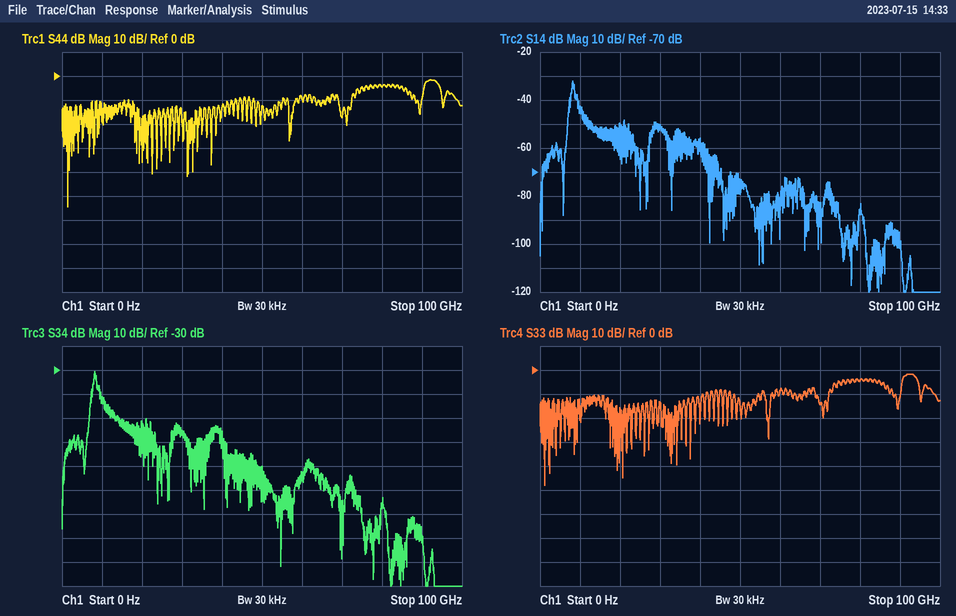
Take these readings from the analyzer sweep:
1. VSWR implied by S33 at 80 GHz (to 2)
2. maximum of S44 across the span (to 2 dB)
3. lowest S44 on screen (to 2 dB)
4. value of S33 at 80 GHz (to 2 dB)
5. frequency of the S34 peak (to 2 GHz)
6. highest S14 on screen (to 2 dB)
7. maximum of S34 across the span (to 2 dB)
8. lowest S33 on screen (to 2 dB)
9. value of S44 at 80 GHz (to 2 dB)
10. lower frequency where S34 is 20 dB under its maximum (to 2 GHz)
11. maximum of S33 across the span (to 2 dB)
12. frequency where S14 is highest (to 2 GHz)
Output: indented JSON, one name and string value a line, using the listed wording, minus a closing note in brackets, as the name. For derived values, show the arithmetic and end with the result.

{
  "VSWR implied by S33 at 80 GHz": "|Γ| = 10^(-4/20) = 0.6310; VSWR = (1 + 0.6310)/(1 − 0.6310) ≈ 4",
  "maximum of S44 across the span": "-2 dB",
  "lowest S44 on screen": "-54 dB",
  "value of S33 at 80 GHz": "-4 dB",
  "frequency of the S34 peak": "8 GHz",
  "highest S14 on screen": "-32 dB",
  "maximum of S34 across the span": "-30 dB",
  "lowest S33 on screen": "-48 dB",
  "value of S44 at 80 GHz": "-4 dB",
  "lower frequency where S34 is 20 dB under its maximum": "6 GHz",
  "maximum of S33 across the span": "-2 dB",
  "frequency where S14 is highest": "8 GHz"
}
